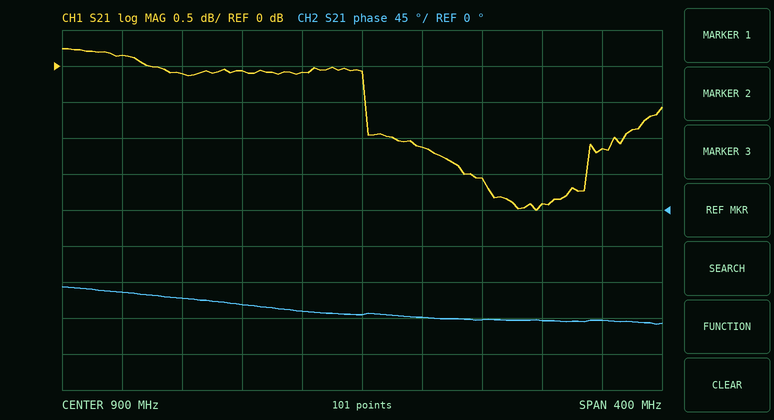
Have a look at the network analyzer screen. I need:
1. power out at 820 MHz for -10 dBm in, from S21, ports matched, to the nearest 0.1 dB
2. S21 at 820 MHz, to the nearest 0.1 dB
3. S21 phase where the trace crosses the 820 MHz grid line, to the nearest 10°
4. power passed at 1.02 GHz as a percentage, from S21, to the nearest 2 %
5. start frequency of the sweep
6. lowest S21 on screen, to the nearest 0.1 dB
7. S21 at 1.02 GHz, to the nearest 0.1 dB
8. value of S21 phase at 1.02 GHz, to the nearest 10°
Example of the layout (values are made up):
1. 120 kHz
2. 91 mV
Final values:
1. -10.1 dBm
2. -0.1 dB
3. -120°
4. 64 %
5. 700 MHz
6. -2.0 dB
7. -1.9 dB
8. -140°
